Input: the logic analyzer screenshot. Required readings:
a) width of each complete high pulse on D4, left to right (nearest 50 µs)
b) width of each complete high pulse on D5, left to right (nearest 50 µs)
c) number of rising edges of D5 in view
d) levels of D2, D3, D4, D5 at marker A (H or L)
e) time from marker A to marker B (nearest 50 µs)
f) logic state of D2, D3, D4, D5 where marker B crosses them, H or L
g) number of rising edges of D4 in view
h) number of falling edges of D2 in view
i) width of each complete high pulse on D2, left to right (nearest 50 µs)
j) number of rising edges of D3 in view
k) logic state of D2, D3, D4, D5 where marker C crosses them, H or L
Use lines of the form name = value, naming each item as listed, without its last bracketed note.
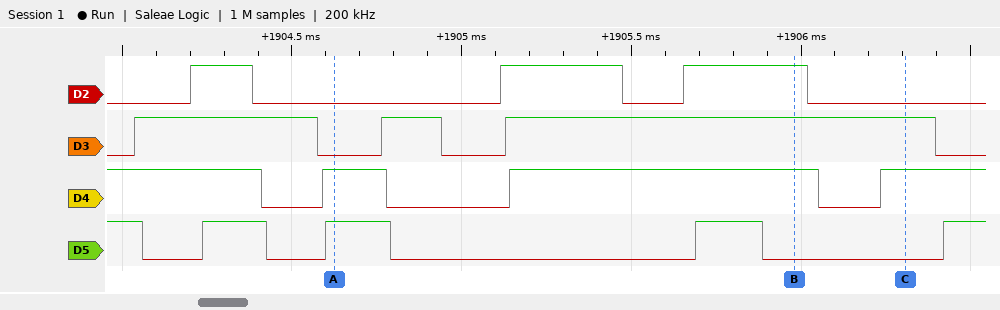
width of each complete high pulse on D4, left to right = 200 µs, 900 µs
width of each complete high pulse on D5, left to right = 200 µs, 200 µs, 200 µs
number of rising edges of D5 in view = 4
levels of D2, D3, D4, D5 at marker A = D2=L, D3=L, D4=H, D5=H
time from marker A to marker B = 1350 µs
logic state of D2, D3, D4, D5 where marker B crosses them, H or L = D2=H, D3=H, D4=H, D5=L
number of rising edges of D4 in view = 3
number of falling edges of D2 in view = 3
width of each complete high pulse on D2, left to right = 200 µs, 350 µs, 350 µs
number of rising edges of D3 in view = 3
logic state of D2, D3, D4, D5 where marker C crosses them, H or L = D2=L, D3=H, D4=H, D5=L
